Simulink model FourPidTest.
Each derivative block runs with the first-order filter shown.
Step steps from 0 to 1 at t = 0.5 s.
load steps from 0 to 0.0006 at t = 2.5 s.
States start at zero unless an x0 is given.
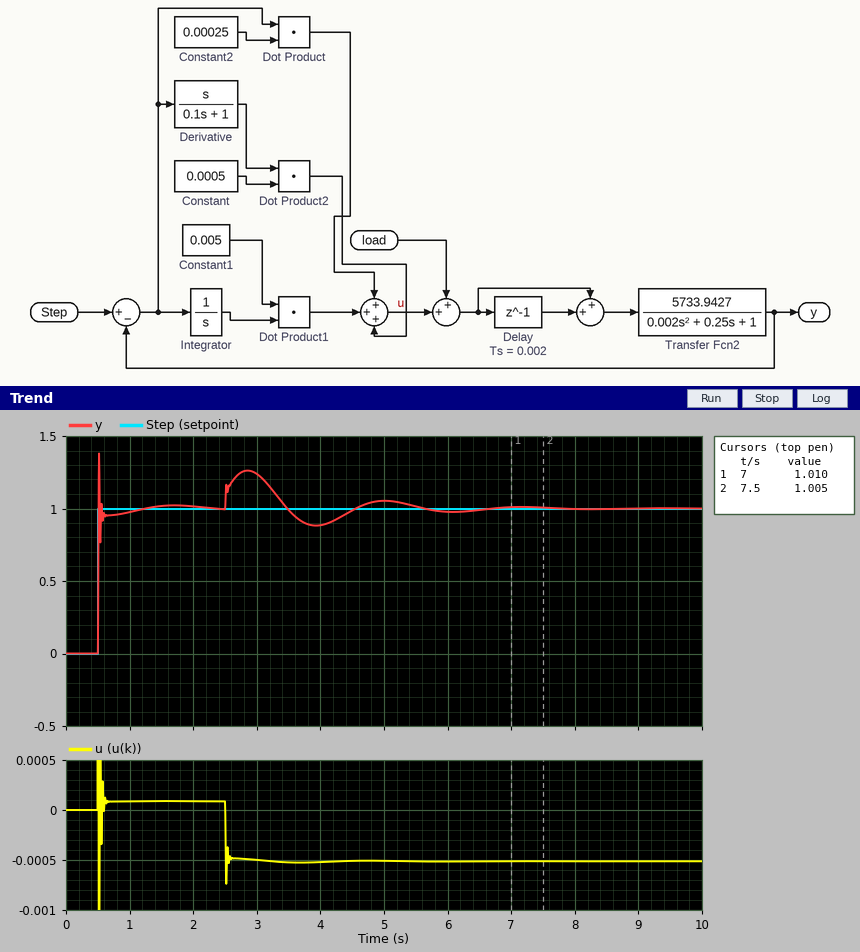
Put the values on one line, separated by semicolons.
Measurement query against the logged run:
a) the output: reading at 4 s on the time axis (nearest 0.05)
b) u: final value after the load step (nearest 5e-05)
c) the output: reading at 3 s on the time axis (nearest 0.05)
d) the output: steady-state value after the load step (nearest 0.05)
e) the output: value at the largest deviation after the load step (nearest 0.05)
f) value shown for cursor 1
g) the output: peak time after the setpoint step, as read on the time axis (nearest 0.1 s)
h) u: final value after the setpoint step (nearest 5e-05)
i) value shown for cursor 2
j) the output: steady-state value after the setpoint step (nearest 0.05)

0.90; -0.00050; 1.25; 1.00; 1.25; 1.010; 0.5 s; 0.00010; 1.005; 1.00
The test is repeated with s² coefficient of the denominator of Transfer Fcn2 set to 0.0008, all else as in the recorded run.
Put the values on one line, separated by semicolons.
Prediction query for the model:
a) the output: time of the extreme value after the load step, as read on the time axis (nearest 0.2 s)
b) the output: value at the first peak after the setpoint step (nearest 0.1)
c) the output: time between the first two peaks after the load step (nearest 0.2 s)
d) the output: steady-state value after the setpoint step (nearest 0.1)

2.8 s; 1.2; 2.2 s; 1.0
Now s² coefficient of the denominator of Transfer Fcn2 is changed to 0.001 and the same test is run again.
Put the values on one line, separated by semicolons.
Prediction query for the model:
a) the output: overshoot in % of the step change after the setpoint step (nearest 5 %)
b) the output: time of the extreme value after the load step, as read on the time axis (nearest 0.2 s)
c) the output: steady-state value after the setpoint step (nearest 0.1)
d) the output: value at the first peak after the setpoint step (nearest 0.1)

25 %; 2.8 s; 1.0; 1.3
